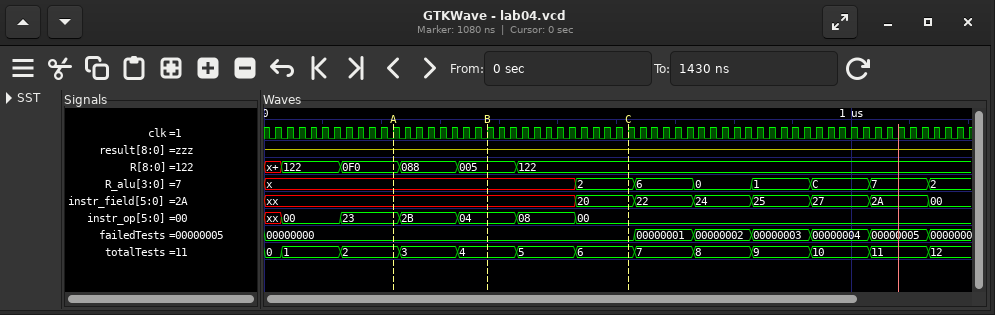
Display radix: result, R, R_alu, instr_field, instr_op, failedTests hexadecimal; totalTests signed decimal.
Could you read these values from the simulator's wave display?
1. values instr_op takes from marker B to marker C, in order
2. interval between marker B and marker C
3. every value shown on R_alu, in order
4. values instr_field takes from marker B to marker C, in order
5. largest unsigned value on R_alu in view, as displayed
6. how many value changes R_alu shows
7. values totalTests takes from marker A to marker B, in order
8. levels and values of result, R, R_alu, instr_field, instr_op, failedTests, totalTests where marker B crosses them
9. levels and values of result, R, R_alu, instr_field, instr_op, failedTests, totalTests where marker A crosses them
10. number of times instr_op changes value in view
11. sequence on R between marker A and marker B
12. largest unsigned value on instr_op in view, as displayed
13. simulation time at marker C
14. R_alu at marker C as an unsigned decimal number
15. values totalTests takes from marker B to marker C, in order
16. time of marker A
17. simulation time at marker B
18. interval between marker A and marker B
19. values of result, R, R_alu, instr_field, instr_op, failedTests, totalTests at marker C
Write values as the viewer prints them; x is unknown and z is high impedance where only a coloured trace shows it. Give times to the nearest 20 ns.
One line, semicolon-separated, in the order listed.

04, 08, 00; 240 ns; x, 2, 6, 0, 1, C, 7, 2; xx, 20; C; 7; 2, 3, 4; result=z, R=005, R_alu=x, instr_field=xx, instr_op=04, failedTests=00000000, totalTests=4; result=z, R=0F0, R_alu=x, instr_field=xx, instr_op=23, failedTests=00000000, totalTests=2; 6; 0F0, 088, 005; 2B; 620 ns; 2; 4, 5, 6; 220 ns; 380 ns; 160 ns; result=z, R=122, R_alu=2, instr_field=20, instr_op=00, failedTests=00000000, totalTests=6
